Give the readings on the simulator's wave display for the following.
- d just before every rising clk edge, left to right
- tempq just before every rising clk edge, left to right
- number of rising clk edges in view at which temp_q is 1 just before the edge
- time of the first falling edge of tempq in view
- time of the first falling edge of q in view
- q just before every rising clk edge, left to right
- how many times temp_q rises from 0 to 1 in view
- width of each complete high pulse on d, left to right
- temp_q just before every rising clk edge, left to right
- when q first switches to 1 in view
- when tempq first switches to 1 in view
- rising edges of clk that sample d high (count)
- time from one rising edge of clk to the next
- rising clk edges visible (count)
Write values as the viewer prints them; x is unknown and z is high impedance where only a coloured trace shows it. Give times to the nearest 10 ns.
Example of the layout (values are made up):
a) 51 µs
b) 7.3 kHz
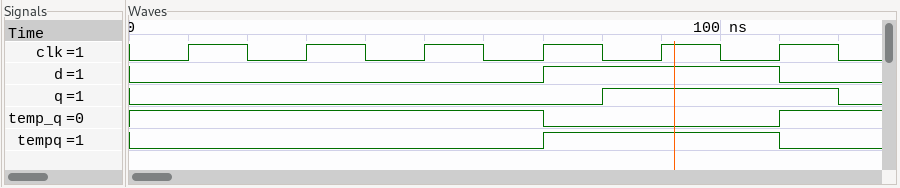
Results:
a) 0 0 0 0 1 1
b) 0 0 0 0 1 1
c) 4
d) 110 ns
e) 120 ns
f) 0 0 0 0 1 1
g) 1
h) 40 ns
i) 1 1 1 1 0 0
j) 80 ns
k) 70 ns
l) 2
m) 20 ns
n) 6
